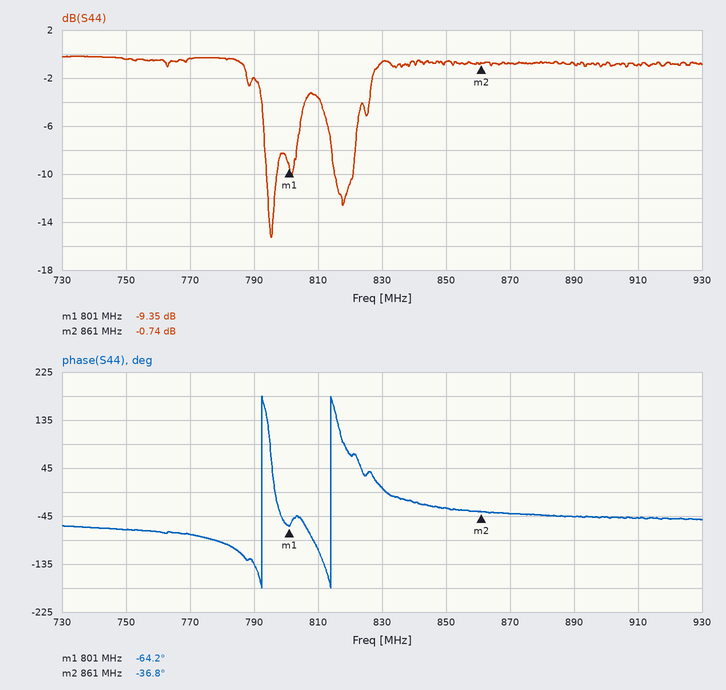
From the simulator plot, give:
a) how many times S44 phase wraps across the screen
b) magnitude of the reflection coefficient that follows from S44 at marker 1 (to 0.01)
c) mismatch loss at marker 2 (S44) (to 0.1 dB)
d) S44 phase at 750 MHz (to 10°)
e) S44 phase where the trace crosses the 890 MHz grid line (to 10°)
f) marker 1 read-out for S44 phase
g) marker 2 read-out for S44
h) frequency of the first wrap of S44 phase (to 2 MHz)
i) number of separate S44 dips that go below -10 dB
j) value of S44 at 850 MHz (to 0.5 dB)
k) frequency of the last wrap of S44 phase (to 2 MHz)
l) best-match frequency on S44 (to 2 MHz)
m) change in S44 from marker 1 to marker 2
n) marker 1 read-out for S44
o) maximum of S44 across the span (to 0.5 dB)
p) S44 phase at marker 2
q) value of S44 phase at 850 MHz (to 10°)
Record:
2
0.34
8.1 dB
-70°
-50°
-64.2°
-0.74 dB
792 MHz
2
-0.5 dB
814 MHz
796 MHz
8.61 dB
-9.35 dB
0.0 dB
-36.8°
-30°
